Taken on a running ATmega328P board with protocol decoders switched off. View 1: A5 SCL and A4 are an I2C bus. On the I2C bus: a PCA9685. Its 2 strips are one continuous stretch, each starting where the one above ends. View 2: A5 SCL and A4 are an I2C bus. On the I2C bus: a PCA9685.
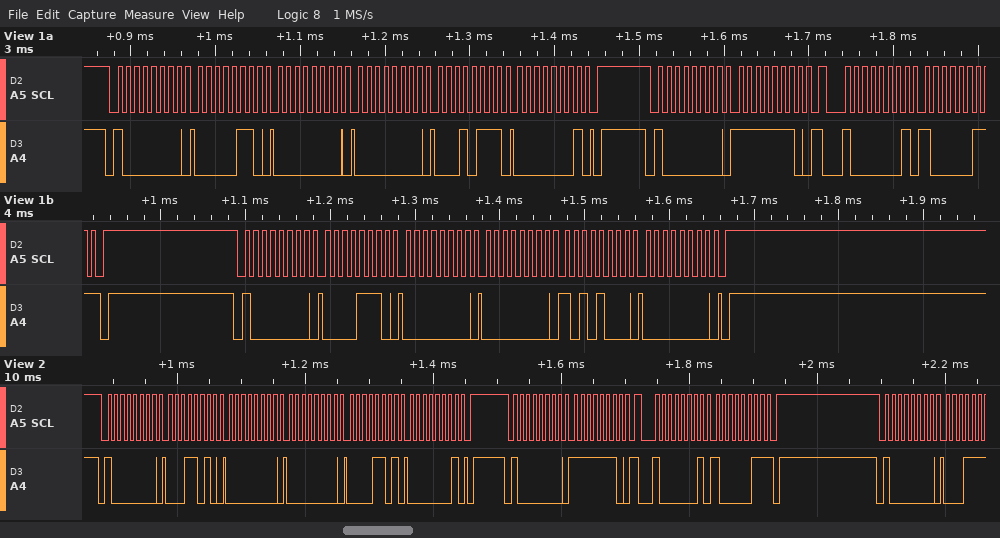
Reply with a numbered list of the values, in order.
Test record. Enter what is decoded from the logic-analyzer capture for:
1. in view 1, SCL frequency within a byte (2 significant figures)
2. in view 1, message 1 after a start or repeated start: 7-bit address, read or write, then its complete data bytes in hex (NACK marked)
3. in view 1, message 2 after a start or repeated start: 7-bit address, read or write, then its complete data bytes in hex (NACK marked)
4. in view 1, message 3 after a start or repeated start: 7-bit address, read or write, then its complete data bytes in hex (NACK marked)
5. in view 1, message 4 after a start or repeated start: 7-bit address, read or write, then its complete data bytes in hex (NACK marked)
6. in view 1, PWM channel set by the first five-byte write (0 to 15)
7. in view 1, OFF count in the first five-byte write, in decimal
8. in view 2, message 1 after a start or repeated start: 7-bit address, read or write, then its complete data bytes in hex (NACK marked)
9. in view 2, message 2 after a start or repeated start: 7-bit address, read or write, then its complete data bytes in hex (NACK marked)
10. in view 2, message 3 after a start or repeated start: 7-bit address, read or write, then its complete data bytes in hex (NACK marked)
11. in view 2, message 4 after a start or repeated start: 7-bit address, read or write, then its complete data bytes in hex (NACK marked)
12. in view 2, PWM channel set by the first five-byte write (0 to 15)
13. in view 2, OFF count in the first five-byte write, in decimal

1. 100 kHz
2. 0x40 write: 06 00 00 17 01
3. 0x40 write: FE
4. 0x40 read: 83 NACK
5. 0x40 write: 0E 00 00 A8 00
6. 0
7. 279
8. 0x40 write: 1A 00 00 0D 01
9. 0x40 write: FE
10. 0x40 read: 83 NACK
11. 0x40 write
12. 5
13. 269
